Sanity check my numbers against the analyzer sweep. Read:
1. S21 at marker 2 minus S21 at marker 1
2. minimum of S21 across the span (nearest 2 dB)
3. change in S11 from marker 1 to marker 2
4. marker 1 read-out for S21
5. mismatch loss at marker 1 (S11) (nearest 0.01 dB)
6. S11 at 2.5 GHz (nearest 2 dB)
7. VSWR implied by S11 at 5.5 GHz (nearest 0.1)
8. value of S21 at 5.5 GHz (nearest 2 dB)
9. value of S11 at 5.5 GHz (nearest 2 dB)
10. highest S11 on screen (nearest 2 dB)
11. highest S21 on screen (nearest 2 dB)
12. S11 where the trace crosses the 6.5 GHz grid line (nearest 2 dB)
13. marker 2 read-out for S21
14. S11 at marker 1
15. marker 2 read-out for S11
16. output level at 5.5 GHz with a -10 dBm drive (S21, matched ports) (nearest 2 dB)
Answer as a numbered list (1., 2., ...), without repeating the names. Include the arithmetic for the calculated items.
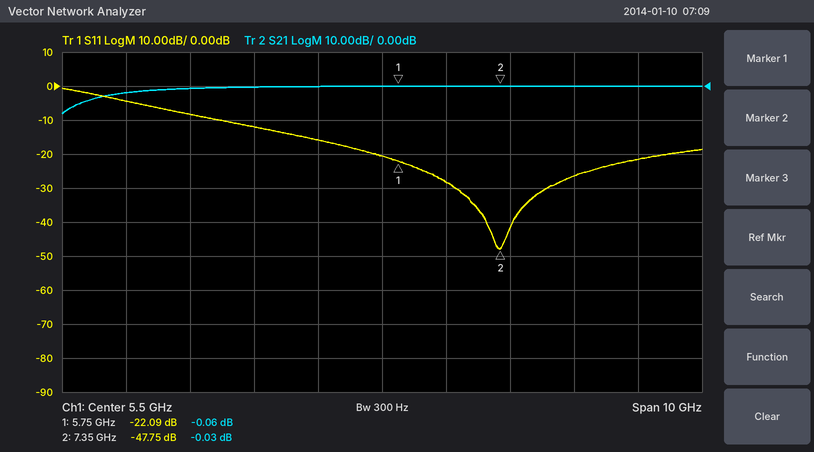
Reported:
1. -0.03 − (-0.06) = 0.03 dB
2. -8 dB
3. -47.75 − (-22.09) = -25.66 dB
4. -0.06 dB
5. −10 log10(1 − 10^(-22.09/10)) ≈ 0.03 dB
6. -8 dB
7. |Γ| = 10^(-20/20) = 0.1000; VSWR = (1 + 0.1000)/(1 − 0.1000) ≈ 1.2
8. 0 dB
9. -20 dB
10. 0 dB
11. 0 dB
12. -28 dB
13. -0.03 dB
14. -22.09 dB
15. -47.75 dB
16. -10 dBm + (0 dB) = -10 dBm
